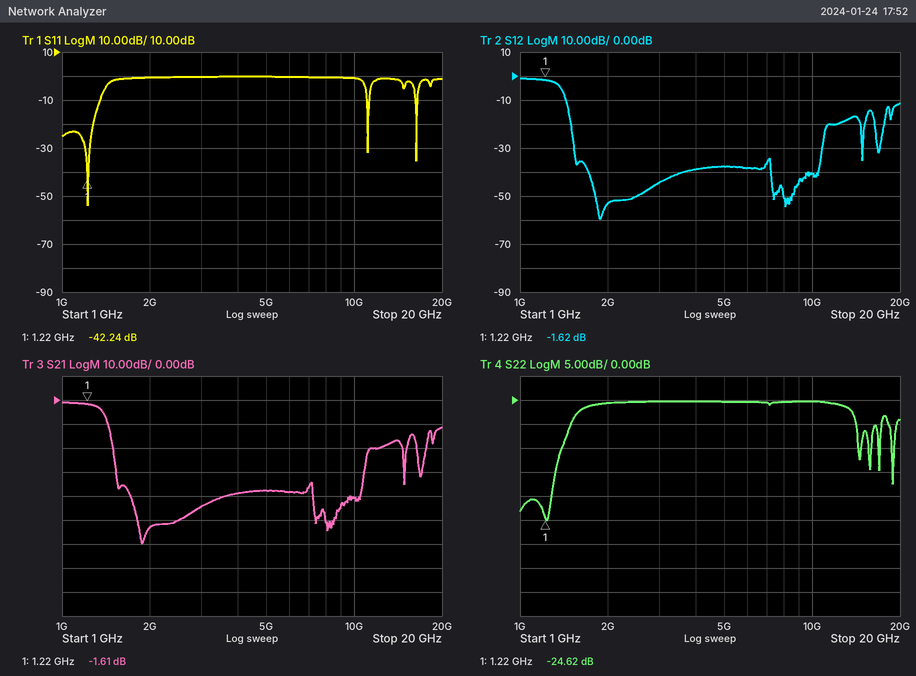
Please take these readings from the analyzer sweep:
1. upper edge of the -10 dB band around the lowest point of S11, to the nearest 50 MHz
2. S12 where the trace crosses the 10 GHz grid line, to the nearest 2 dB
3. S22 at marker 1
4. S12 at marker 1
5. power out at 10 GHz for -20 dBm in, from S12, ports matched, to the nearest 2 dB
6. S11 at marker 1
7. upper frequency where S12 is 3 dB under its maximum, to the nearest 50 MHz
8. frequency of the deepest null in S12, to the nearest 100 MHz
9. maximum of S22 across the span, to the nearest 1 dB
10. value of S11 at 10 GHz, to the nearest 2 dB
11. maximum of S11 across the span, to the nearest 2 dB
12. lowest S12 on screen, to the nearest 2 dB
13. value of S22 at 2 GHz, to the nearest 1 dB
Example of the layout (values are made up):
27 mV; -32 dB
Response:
1.35 GHz; -40 dB; -24.62 dB; -1.62 dB; -60 dBm; -42.24 dB; 1.35 GHz; 1.9 GHz; 0 dB; 0 dB; 0 dB; -60 dB; -1 dB
